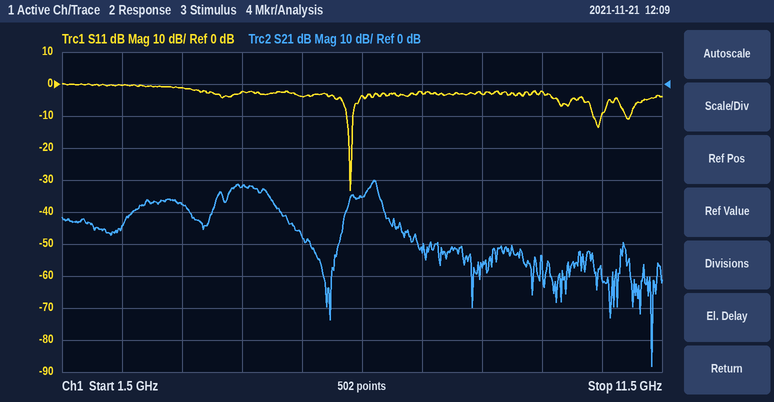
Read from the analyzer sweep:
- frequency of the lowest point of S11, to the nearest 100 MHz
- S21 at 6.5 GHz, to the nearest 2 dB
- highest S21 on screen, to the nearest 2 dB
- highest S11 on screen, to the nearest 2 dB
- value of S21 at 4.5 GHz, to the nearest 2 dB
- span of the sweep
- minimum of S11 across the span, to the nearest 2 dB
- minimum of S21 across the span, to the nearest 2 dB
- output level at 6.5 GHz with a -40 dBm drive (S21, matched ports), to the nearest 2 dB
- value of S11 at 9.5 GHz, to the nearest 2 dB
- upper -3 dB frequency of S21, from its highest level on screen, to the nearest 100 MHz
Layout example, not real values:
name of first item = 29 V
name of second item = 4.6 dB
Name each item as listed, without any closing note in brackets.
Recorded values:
frequency of the lowest point of S11, to the nearest 100 MHz = 6.3 GHz
S21 at 6.5 GHz, to the nearest 2 dB = -36 dB
highest S21 on screen, to the nearest 2 dB = -30 dB
highest S11 on screen, to the nearest 2 dB = 0 dB
value of S21 at 4.5 GHz, to the nearest 2 dB = -32 dB
span of the sweep = 10 GHz
minimum of S11 across the span, to the nearest 2 dB = -34 dB
minimum of S21 across the span, to the nearest 2 dB = -88 dB
output level at 6.5 GHz with a -40 dBm drive (S21, matched ports), to the nearest 2 dB = -76 dBm
value of S11 at 9.5 GHz, to the nearest 2 dB = -2 dB
upper -3 dB frequency of S21, from its highest level on screen, to the nearest 100 MHz = 6.8 GHz
